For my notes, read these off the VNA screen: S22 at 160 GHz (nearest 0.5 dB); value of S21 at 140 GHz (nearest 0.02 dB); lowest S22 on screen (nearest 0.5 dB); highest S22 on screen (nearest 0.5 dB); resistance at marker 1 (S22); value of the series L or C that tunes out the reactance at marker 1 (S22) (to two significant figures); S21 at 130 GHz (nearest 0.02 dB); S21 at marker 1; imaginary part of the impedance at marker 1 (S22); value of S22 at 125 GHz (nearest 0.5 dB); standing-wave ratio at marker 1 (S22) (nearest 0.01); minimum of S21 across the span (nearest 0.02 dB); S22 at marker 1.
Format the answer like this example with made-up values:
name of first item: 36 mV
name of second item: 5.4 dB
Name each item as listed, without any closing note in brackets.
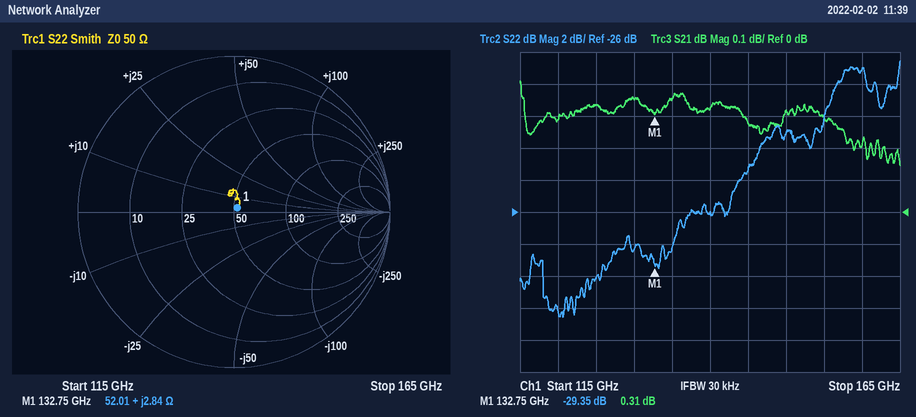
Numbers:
S22 at 160 GHz: -17.0 dB
value of S21 at 140 GHz: 0.32 dB
lowest S22 on screen: -32.5 dB
highest S22 on screen: -16.5 dB
resistance at marker 1: 52.01 Ω
value of the series L or C that tunes out the reactance at marker 1 (S22): 420 fF
S21 at 130 GHz: 0.36 dB
S21 at marker 1: 0.31 dB
imaginary part of the impedance at marker 1: +2.84 Ω
value of S22 at 125 GHz: -30.0 dB
standing-wave ratio at marker 1 (S22): 1.07
minimum of S21 across the span: 0.14 dB
S22 at marker 1: -29.35 dB
